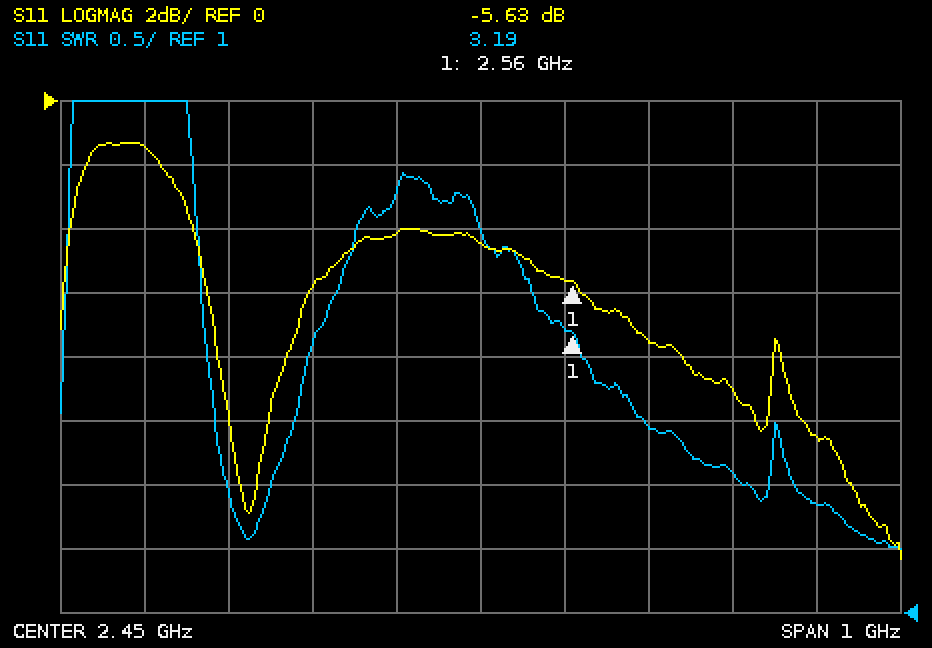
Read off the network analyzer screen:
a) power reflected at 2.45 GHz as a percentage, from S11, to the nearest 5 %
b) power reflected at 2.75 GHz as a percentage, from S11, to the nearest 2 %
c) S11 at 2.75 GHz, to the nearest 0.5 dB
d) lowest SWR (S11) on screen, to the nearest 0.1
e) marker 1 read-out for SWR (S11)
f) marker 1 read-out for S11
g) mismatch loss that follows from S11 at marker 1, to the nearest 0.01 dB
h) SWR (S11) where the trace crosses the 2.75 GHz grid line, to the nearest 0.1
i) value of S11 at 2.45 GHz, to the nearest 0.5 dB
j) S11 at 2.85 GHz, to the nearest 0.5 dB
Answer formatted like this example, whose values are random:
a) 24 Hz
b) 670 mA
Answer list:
a) 35 %
b) 12 %
c) -9.0 dB
d) 1.5
e) 3.19
f) -5.63 dB
g) 1.39 dB
h) 2.1
i) -4.5 dB
j) -10.5 dB
